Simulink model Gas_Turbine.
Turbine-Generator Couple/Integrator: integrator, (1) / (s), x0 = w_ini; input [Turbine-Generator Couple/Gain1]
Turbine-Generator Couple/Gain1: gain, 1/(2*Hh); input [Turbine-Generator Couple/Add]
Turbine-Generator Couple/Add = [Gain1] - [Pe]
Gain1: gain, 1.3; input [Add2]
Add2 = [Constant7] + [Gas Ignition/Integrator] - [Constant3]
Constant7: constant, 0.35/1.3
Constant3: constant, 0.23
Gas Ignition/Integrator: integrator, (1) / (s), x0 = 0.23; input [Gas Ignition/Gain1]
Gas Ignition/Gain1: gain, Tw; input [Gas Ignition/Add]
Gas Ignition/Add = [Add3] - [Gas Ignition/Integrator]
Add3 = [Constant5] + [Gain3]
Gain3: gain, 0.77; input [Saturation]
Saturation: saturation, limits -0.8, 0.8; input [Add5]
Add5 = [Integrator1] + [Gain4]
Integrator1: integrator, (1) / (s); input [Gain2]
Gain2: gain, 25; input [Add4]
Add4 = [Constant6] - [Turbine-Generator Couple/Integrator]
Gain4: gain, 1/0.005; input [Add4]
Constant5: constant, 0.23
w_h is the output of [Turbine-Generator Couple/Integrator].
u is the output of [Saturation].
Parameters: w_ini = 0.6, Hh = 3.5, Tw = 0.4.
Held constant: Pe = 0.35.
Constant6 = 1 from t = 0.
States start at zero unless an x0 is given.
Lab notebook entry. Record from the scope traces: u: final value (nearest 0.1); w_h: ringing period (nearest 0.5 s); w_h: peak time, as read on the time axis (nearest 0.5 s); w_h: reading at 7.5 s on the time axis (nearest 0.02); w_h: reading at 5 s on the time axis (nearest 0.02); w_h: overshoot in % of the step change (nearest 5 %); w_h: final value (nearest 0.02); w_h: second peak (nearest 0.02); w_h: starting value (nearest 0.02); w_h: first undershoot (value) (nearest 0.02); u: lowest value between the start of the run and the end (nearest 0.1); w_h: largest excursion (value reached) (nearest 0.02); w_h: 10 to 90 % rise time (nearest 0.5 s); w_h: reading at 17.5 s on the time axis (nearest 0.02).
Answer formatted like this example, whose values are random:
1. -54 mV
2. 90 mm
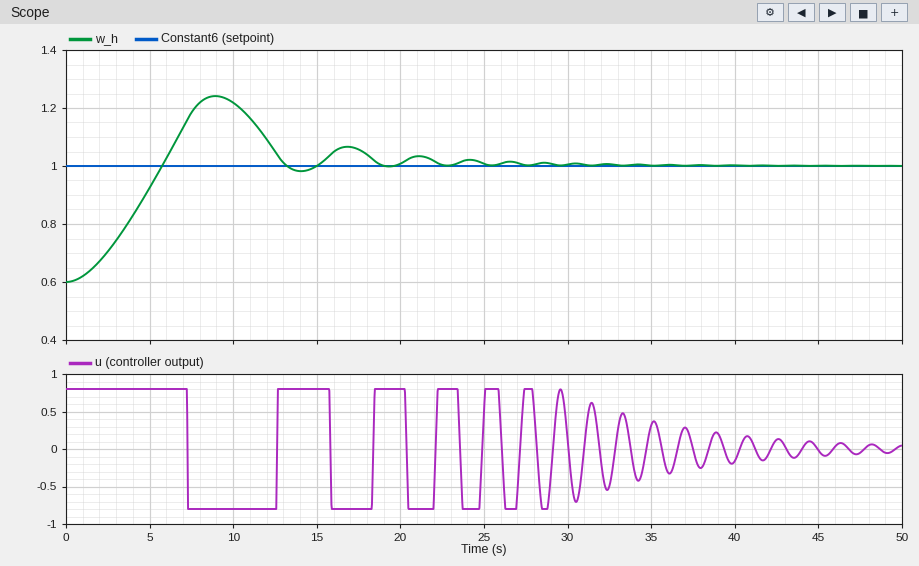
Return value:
1. 0.0
2. 8.0 s
3. 9.0 s
4. 1.18
5. 0.92
6. 60 %
7. 1.00
8. 1.06
9. 0.60
10. 0.98
11. -0.8
12. 1.24
13. 4.0 s
14. 1.06
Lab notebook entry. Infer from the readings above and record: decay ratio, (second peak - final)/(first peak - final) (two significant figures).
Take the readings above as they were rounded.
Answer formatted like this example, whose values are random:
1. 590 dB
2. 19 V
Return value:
1. 0.25
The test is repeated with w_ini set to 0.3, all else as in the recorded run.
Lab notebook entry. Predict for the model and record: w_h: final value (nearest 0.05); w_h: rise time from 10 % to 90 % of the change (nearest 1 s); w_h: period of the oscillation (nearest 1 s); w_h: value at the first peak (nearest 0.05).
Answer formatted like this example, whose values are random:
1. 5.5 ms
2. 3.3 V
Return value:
1. 1.00
2. 6 s
3. 10 s
4. 1.45
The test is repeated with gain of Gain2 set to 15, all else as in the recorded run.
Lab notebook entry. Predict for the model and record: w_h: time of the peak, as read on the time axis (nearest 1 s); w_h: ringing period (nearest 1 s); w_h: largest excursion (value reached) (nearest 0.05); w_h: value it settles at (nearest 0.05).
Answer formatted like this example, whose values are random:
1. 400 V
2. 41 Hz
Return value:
1. 8 s
2. 6 s
3. 1.20
4. 1.00
